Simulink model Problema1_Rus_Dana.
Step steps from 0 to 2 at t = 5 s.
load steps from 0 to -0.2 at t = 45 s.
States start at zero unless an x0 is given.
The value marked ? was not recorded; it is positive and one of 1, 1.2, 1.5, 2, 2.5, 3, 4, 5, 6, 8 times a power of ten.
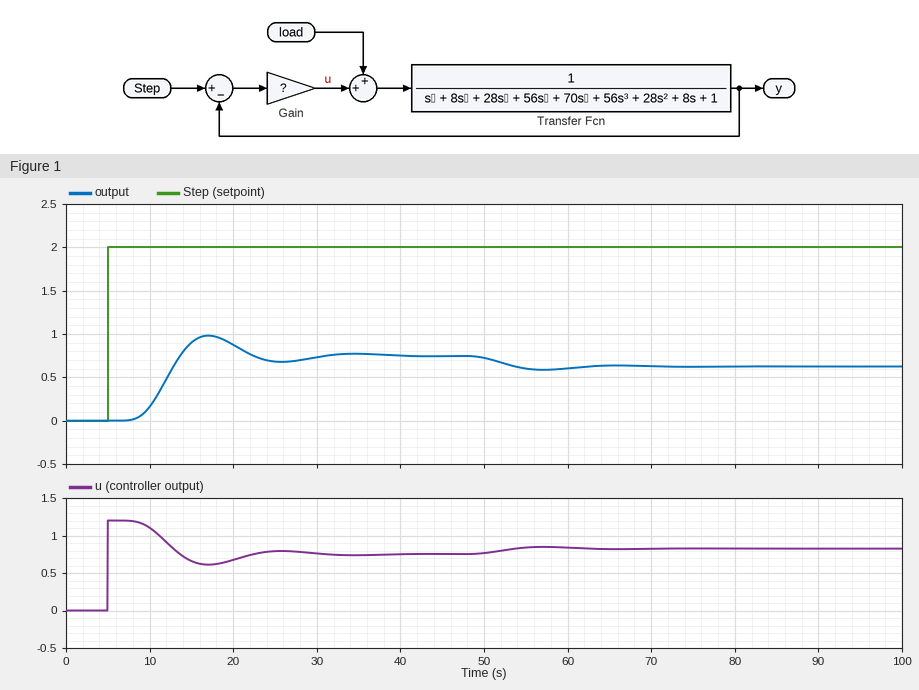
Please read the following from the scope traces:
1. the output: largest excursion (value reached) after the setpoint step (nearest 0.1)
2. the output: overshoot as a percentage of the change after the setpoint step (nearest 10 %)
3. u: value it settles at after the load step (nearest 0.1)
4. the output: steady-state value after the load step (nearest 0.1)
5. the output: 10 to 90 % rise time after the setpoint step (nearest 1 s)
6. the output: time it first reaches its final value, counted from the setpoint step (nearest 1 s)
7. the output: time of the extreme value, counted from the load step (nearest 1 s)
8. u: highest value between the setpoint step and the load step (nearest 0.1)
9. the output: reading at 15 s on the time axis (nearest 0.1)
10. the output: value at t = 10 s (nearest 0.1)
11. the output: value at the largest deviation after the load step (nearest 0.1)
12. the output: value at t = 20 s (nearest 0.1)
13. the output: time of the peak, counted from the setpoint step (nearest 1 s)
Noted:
1.0
30 %
0.8
0.6
4 s
9 s
12 s
1.2
0.9
0.2
0.6
0.9
12 s
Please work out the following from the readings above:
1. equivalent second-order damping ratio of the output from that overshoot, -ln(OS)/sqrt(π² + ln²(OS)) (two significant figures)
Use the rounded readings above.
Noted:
0.36
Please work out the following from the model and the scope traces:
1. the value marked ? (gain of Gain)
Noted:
0.6
